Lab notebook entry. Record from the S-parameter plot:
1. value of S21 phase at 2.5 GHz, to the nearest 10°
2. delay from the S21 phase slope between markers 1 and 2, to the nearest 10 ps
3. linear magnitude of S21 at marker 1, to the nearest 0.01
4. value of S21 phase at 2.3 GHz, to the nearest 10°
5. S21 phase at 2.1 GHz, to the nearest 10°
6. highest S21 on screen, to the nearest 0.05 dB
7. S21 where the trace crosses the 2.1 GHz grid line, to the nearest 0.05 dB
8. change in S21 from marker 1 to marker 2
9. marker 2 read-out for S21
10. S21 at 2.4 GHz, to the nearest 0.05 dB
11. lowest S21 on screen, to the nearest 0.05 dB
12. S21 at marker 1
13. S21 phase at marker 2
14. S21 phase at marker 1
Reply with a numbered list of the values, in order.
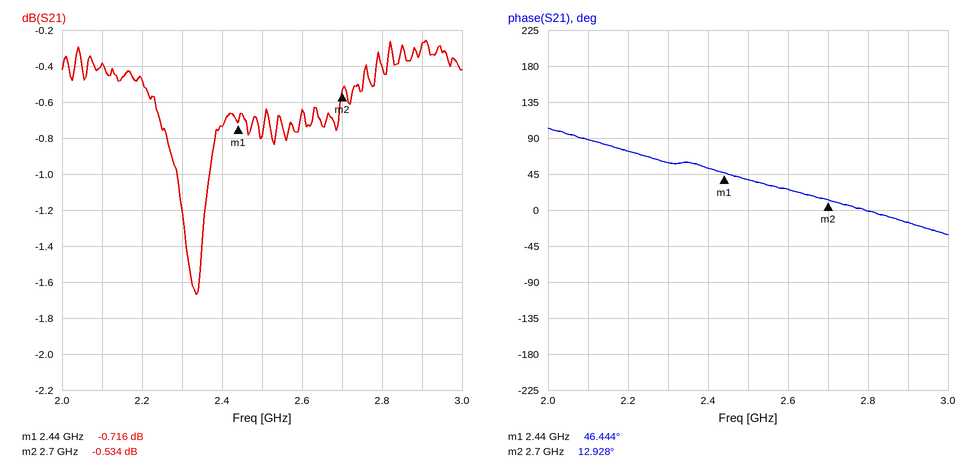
1. 40°
2. 360 ps
3. 0.92
4. 60°
5. 90°
6. -0.25 dB
7. -0.40 dB
8. 0.182 dB
9. -0.534 dB
10. -0.75 dB
11. -1.65 dB
12. -0.716 dB
13. 12.928°
14. 46.444°
